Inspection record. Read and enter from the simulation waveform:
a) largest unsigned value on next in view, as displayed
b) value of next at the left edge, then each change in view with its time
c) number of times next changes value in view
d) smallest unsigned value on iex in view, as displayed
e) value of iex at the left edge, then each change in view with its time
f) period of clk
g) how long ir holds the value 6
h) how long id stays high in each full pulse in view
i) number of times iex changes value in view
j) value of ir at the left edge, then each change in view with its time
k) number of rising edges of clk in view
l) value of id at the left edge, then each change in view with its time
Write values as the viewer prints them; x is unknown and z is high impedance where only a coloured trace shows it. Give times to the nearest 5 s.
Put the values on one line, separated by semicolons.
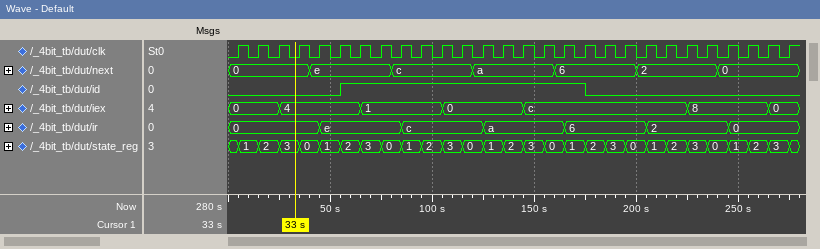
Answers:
e; 0, e at 40 s, c at 80 s, a at 120 s, 6 at 160 s, 2 at 200 s, 0 at 240 s; 6; 0; 0, 4 at 25 s, 1 at 65 s, 0 at 105 s, c at 145 s, 8 at 225 s, 0 at 265 s; 10 s; 40 s; 120 s; 6; 0, e at 45 s, c at 85 s, a at 125 s, 6 at 165 s, 2 at 205 s, 0 at 245 s; 28; 0, 1 at 55 s, 0 at 175 s
